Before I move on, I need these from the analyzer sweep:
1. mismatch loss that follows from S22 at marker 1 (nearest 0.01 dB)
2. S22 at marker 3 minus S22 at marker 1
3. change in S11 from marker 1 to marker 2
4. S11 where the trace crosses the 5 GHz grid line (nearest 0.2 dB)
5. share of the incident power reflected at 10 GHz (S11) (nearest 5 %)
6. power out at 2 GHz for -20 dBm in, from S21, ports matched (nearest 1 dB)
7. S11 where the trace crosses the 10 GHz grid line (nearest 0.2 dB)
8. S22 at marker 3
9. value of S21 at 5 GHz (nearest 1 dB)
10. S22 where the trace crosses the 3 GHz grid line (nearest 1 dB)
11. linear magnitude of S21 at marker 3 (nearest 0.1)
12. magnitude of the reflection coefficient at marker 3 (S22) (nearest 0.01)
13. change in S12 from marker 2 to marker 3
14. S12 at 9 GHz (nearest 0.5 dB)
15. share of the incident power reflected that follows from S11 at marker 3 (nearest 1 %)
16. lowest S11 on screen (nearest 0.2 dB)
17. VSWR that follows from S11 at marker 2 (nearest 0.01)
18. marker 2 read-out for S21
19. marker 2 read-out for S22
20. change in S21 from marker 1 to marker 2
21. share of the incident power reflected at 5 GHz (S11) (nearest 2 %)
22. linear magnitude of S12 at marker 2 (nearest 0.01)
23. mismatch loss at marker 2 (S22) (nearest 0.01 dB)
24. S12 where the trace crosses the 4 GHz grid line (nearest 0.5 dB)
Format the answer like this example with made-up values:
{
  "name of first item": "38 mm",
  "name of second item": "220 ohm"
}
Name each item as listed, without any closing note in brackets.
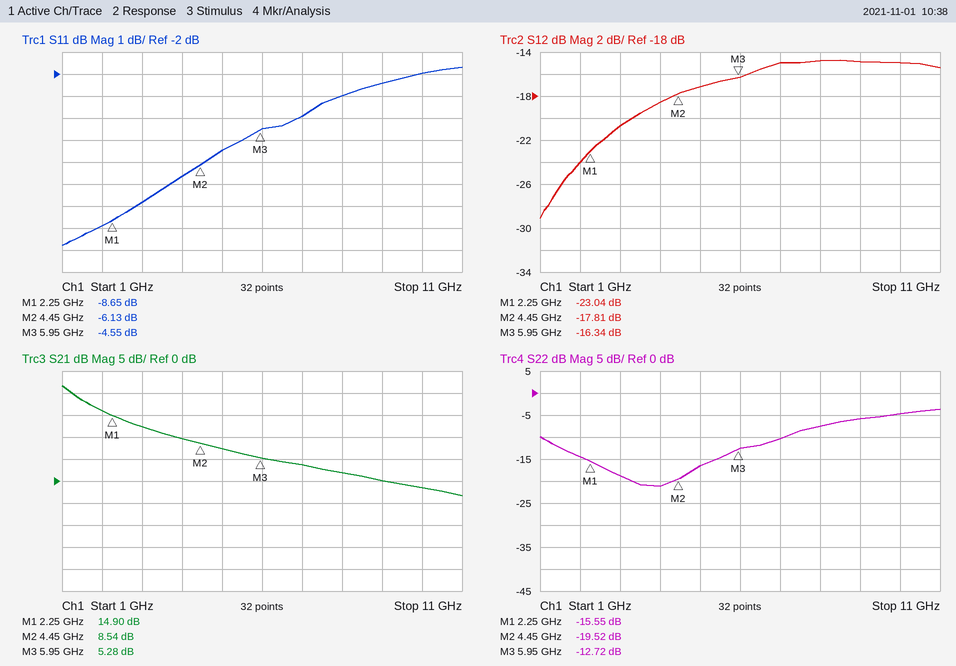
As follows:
{
  "mismatch loss that follows from S22 at marker 1": "0.12 dB",
  "S22 at marker 3 minus S22 at marker 1": "2.83 dB",
  "change in S11 from marker 1 to marker 2": "2.52 dB",
  "S11 where the trace crosses the 5 GHz grid line": "-5.4 dB",
  "share of the incident power reflected at 10 GHz (S11)": "65 %",
  "power out at 2 GHz for -20 dBm in, from S21, ports matched": "-4 dBm",
  "S11 where the trace crosses the 10 GHz grid line": "-2.0 dB",
  "S22 at marker 3": "-12.72 dB",
  "value of S21 at 5 GHz": "7 dB",
  "S22 where the trace crosses the 3 GHz grid line": "-19 dB",
  "linear magnitude of S21 at marker 3": "1.8",
  "magnitude of the reflection coefficient at marker 3 (S22)": "0.23",
  "change in S12 from marker 2 to marker 3": "1.47 dB",
  "S12 at 9 GHz": "-15.0 dB",
  "share of the incident power reflected that follows from S11 at marker 3": "35 %",
  "lowest S11 on screen": "-9.8 dB",
  "VSWR that follows from S11 at marker 2": "2.95",
  "marker 2 read-out for S21": "8.54 dB",
  "marker 2 read-out for S22": "-19.52 dB",
  "change in S21 from marker 1 to marker 2": "-6.36 dB",
  "share of the incident power reflected at 5 GHz (S11)": "28 %",
  "linear magnitude of S12 at marker 2": "0.13",
  "mismatch loss at marker 2 (S22)": "0.05 dB",
  "S12 where the trace crosses the 4 GHz grid line": "-18.5 dB"
}
